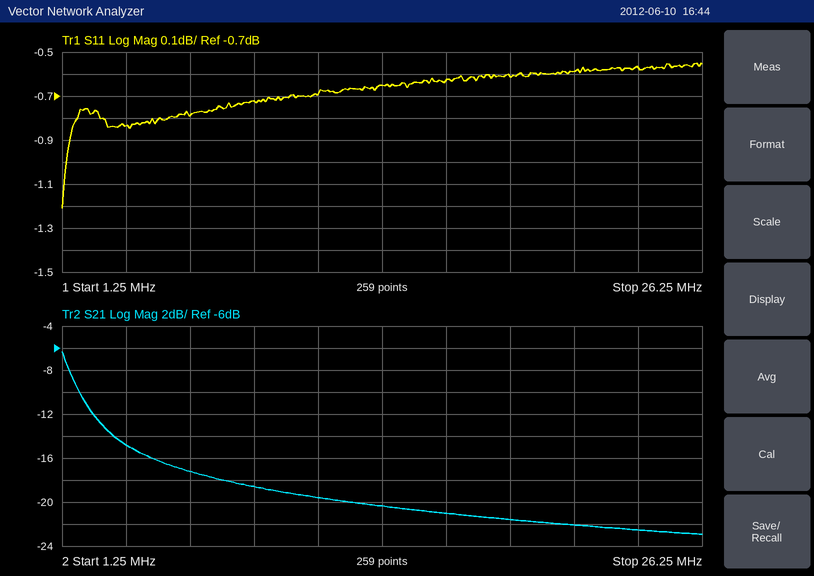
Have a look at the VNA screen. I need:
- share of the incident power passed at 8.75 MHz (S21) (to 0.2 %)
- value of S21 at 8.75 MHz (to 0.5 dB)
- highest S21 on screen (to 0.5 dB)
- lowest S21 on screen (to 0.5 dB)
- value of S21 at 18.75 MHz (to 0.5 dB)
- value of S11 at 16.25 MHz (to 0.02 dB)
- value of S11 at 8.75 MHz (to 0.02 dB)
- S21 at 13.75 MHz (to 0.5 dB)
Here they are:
1.4 %
-18.5 dB
-6.5 dB
-23.0 dB
-21.5 dB
-0.62 dB
-0.72 dB
-20.5 dB
